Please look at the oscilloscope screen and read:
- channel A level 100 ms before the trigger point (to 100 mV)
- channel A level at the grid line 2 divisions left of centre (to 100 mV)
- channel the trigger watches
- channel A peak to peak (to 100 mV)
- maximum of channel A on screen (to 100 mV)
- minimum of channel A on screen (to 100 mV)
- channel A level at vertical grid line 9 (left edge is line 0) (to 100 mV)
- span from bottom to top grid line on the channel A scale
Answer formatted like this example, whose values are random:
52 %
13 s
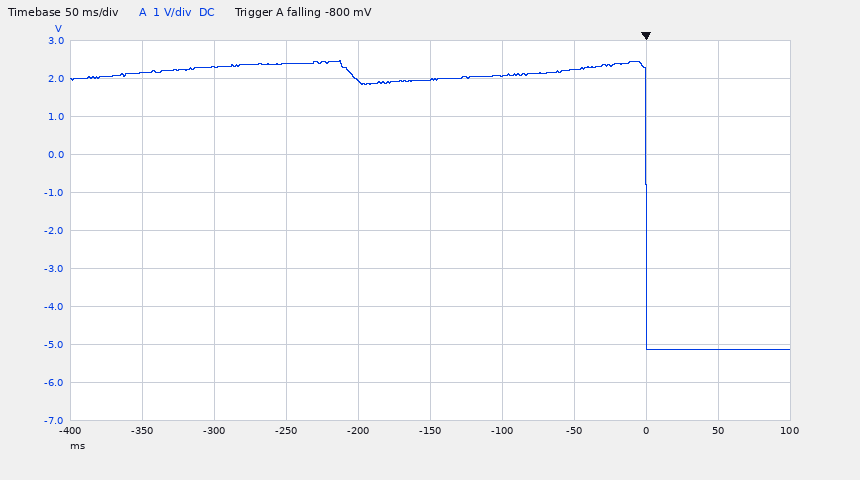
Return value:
2.1 V
2.4 V
channel A
7.6 V
2.5 V
-5.1 V
-5.1 V
10 V
